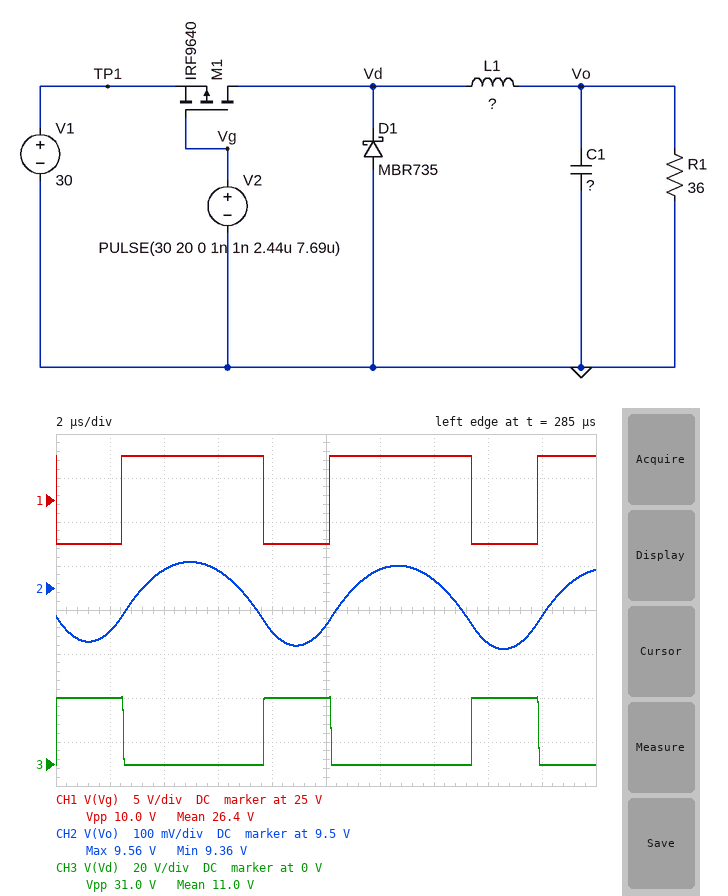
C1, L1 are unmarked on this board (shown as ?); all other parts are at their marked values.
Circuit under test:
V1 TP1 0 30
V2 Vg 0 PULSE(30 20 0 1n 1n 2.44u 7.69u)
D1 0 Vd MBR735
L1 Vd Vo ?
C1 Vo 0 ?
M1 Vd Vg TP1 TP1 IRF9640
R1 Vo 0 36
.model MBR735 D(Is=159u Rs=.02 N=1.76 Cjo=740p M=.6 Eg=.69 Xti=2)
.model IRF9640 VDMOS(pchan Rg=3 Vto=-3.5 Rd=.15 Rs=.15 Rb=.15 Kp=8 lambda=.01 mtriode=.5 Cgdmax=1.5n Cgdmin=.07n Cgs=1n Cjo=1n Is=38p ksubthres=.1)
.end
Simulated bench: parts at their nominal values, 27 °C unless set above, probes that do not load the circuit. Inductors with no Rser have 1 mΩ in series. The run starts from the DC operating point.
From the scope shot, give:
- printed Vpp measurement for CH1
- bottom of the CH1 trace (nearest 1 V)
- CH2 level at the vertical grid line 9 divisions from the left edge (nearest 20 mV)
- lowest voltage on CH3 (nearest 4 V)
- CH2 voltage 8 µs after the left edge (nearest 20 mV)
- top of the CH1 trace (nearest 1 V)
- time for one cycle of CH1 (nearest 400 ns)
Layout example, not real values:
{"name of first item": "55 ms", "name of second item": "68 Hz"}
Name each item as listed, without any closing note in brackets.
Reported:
{"printed Vpp measurement for CH1": "10.0 V", "bottom of the CH1 trace": "20 V", "CH2 level at the vertical grid line 9 divisions from the left edge": "9.44 V", "lowest voltage on CH3": "0 V", "CH2 voltage 8 µs after the left edge": "9.40 V", "top of the CH1 trace": "30 V", "time for one cycle of CH1": "7.6 µs"}
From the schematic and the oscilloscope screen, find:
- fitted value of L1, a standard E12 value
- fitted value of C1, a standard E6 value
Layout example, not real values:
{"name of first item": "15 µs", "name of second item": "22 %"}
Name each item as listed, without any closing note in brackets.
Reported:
{"fitted value of L1, a standard E12 value": "390 µH", "fitted value of C1, a standard E6 value": "680 nF"}
